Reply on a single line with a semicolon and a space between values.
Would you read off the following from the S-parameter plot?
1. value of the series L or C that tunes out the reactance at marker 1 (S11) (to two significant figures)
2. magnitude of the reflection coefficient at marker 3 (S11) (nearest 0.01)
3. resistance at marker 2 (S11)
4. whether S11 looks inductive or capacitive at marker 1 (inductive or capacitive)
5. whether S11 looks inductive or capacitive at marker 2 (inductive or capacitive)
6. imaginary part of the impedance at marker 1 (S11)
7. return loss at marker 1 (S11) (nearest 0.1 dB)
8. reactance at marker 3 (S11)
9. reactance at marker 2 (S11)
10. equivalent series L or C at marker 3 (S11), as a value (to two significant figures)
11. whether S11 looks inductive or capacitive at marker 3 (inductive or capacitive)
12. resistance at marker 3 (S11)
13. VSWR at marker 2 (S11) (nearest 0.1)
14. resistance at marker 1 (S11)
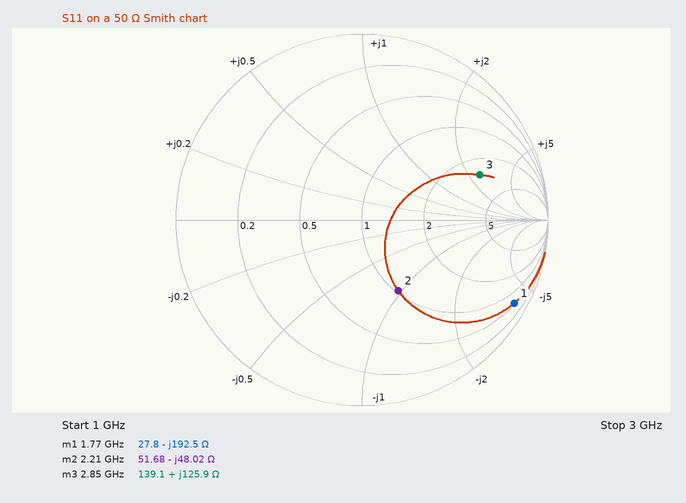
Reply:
17 nH; 0.68; 51.68 Ω; capacitive; capacitive; -192.5 Ω; 0.6 dB; +125.9 Ω; -48.02 Ω; 7.0 nH; inductive; 139.1 Ω; 2.5; 27.8 Ω
